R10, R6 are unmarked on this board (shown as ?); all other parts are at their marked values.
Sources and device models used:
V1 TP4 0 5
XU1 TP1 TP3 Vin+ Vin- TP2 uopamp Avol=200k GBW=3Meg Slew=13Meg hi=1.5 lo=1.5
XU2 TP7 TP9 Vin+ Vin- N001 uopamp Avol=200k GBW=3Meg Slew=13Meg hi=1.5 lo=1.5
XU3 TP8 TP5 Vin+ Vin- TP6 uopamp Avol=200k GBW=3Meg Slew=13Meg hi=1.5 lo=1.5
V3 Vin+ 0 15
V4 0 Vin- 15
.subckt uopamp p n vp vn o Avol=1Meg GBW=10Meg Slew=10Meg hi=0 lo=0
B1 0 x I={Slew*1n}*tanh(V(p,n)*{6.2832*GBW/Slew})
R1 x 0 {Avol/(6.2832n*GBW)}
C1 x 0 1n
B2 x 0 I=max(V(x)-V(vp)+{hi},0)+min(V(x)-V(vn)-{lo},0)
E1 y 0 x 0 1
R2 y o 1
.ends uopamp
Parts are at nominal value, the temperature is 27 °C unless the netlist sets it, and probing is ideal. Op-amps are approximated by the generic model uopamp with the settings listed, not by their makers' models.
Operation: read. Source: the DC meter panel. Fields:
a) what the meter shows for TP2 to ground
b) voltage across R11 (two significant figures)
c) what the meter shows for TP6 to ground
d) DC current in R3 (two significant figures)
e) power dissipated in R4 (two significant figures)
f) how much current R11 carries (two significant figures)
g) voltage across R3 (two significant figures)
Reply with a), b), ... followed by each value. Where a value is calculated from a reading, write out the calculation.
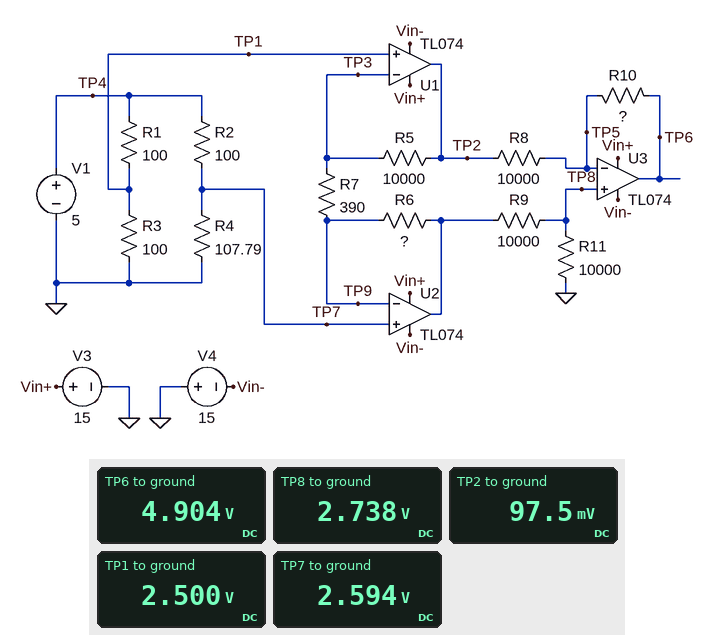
a) 97.5 mV
b) 2.738 V = 2.7 V
c) 4.904 V
d) (2.5 V) / 100 Ω = 25 mA
e) (2.594 V)^2 / 107.8 Ω = 62 mW
f) (2.738 V) / 10 kΩ = 270 µA
g) 2.5 V = 2.5 V
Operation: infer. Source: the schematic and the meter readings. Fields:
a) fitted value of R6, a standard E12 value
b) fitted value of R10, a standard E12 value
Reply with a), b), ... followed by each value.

a) 12 kΩ
b) 8.2 kΩ
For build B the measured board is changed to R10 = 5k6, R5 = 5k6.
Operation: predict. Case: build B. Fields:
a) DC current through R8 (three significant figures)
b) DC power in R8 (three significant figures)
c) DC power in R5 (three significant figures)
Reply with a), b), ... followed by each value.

a) 158 µA
b) 251 µW
c) 323 µW
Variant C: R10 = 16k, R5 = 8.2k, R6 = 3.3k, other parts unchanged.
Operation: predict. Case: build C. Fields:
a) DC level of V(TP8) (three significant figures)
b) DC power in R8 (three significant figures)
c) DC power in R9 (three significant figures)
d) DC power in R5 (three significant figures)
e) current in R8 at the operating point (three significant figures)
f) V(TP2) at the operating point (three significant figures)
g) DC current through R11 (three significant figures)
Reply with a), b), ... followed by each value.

a) 1.69 V
b) 135 µW
c) 287 µW
d) 473 µW
e) 116 µA
f) 530 mV
g) 169 µA
